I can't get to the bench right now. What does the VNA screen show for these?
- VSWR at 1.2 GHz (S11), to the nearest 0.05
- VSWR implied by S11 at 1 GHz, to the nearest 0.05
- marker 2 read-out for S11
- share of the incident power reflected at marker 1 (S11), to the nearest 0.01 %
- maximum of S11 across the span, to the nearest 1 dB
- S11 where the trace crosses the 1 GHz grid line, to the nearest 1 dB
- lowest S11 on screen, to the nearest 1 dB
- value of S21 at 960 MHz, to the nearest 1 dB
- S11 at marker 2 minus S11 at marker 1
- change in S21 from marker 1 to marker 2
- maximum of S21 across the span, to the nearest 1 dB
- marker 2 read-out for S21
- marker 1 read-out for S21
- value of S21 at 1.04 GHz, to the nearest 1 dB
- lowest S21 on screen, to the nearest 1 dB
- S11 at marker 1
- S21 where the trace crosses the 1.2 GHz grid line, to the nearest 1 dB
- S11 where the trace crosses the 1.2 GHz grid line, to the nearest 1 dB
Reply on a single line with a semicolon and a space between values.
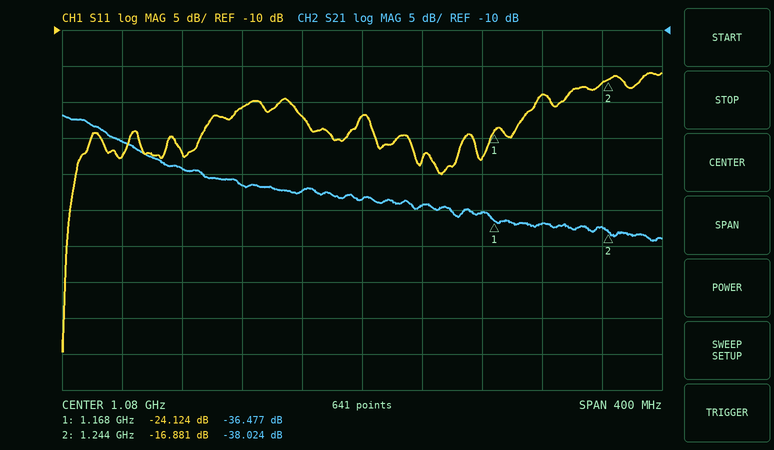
1.25; 1.20; -16.881 dB; 0.39 %; -16 dB; -21 dB; -55 dB; -29 dB; 7.243 dB; -1.547 dB; -22 dB; -38.024 dB; -36.477 dB; -32 dB; -39 dB; -24.124 dB; -37 dB; -19 dB
